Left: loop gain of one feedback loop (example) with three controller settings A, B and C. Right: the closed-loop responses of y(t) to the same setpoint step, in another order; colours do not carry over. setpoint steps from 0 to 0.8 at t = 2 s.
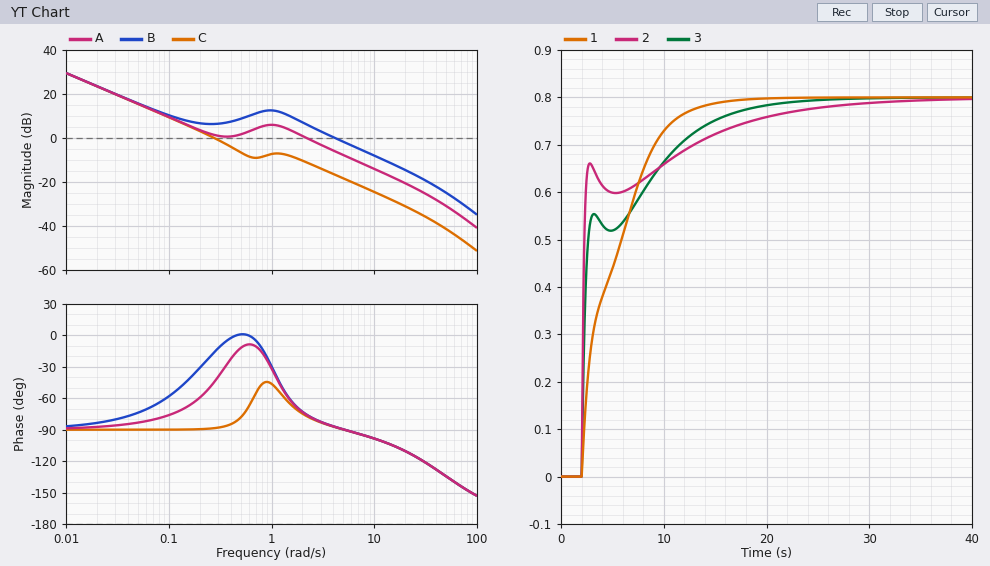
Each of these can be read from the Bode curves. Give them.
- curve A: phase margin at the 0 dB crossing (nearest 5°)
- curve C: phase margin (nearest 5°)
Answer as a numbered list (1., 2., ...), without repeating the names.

1. 105°
2. 90°
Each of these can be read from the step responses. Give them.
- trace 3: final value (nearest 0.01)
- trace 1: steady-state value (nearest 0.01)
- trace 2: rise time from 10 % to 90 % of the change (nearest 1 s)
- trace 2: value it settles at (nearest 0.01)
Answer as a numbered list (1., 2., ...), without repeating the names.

1. 0.80
2. 0.80
3. 13 s
4. 0.80
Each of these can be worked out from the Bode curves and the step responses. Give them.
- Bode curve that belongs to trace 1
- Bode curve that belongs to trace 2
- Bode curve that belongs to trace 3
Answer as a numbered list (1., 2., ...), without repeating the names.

1. C
2. B
3. A
